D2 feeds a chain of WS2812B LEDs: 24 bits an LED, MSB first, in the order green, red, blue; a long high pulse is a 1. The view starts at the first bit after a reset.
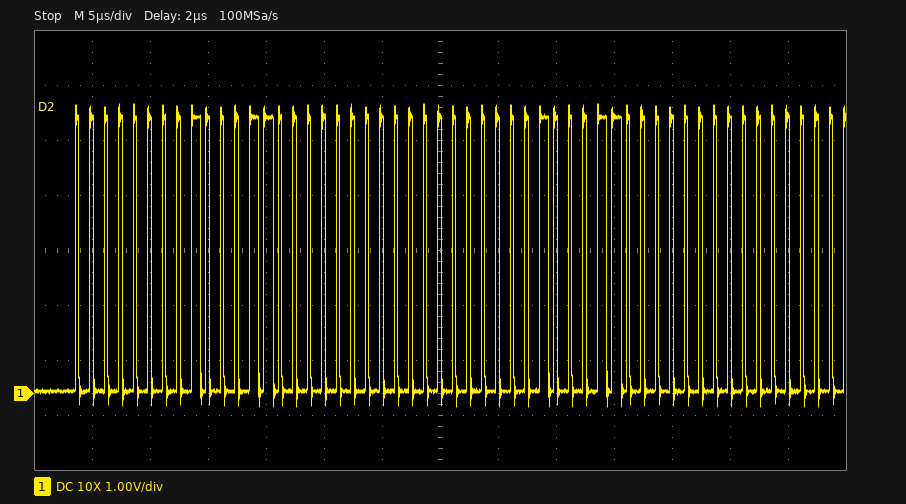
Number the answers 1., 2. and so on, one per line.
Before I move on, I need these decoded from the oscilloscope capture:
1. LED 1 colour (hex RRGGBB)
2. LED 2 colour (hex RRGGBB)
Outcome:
1. #8C0000
2. #8C0000
